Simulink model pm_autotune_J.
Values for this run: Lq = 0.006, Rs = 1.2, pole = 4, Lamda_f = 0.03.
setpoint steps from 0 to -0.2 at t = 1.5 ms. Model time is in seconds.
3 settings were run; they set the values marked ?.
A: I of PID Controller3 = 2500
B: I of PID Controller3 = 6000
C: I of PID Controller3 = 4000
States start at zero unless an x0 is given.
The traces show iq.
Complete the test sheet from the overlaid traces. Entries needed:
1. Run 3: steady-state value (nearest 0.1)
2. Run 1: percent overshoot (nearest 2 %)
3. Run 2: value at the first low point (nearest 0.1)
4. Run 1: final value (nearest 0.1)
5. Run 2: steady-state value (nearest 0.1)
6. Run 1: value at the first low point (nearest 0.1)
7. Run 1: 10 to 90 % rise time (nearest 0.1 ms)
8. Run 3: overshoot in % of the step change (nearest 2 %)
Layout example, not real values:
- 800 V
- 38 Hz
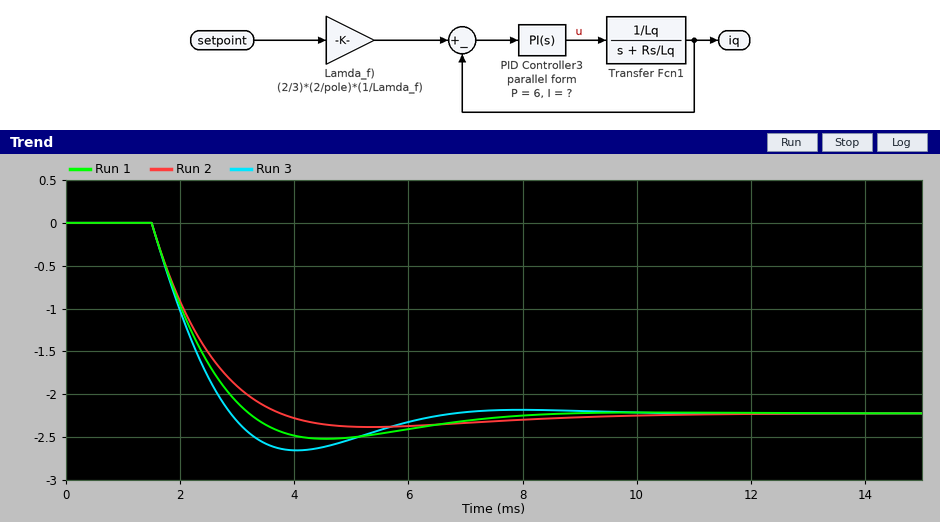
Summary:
- -2.2
- 14 %
- -2.4
- -2.2
- -2.2
- -2.5
- 1.3 ms
- 20 %
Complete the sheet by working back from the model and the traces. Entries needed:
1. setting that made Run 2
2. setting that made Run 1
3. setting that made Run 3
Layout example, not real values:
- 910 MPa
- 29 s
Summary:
- A
- C
- B
